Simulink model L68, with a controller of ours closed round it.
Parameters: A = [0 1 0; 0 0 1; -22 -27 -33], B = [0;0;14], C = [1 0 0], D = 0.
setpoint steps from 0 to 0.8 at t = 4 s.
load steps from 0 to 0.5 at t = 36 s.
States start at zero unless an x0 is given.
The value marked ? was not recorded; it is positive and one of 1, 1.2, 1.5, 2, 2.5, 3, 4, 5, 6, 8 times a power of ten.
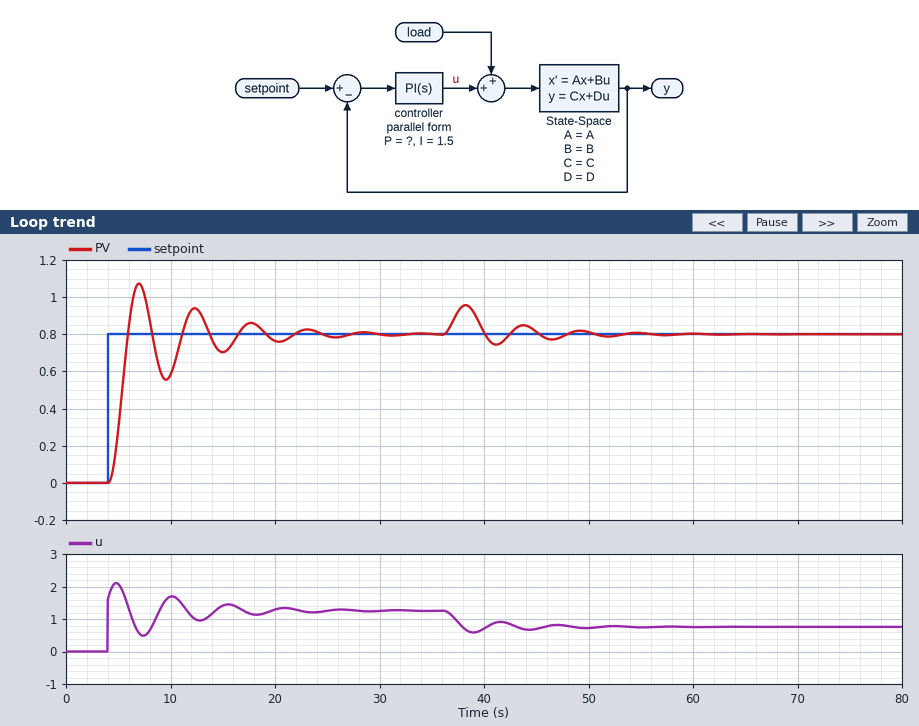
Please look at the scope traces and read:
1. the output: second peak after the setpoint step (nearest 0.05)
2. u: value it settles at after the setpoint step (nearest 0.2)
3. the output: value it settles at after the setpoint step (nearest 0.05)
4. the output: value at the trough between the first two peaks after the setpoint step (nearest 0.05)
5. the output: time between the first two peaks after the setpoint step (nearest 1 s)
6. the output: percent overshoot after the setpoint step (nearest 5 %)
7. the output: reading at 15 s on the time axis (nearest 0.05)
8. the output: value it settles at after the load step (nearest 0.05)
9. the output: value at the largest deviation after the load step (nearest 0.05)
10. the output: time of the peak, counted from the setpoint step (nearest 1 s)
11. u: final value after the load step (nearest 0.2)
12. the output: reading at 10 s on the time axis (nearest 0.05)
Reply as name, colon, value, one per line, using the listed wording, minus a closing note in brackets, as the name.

the output: second peak after the setpoint step: 0.95
u: value it settles at after the setpoint step: 1.2
the output: value it settles at after the setpoint step: 0.80
the output: value at the trough between the first two peaks after the setpoint step: 0.55
the output: time between the first two peaks after the setpoint step: 5 s
the output: percent overshoot after the setpoint step: 35 %
the output: reading at 15 s on the time axis: 0.70
the output: value it settles at after the load step: 0.80
the output: value at the largest deviation after the load step: 0.95
the output: time of the peak, counted from the setpoint step: 3 s
u: final value after the load step: 0.8
the output: reading at 10 s on the time axis: 0.60
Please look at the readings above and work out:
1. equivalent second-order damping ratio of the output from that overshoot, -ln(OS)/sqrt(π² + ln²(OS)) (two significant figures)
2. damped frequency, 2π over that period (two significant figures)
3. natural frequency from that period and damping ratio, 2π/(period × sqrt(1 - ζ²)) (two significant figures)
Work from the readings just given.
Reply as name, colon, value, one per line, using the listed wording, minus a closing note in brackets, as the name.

equivalent second-order damping ratio of the output from that overshoot, -ln(OS)/sqrt(π² + ln²(OS)): 0.32
damped frequency, 2π over that period: 1.3 rad/s
natural frequency from that period and damping ratio, 2π/(period × sqrt(1 - ζ²)): 1.3 rad/s
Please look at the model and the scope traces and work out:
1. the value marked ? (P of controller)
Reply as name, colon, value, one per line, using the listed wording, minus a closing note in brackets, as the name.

the value marked ?: 2
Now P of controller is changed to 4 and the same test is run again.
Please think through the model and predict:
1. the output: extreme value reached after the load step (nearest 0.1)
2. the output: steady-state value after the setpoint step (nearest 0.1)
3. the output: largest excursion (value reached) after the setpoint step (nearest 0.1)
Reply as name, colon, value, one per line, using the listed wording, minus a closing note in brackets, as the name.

the output: extreme value reached after the load step: 0.9
the output: steady-state value after the setpoint step: 0.8
the output: largest excursion (value reached) after the setpoint step: 1.1
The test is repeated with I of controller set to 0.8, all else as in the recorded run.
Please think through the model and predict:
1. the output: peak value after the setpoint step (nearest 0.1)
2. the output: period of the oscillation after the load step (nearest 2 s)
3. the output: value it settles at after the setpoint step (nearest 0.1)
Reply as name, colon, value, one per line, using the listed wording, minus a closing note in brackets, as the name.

the output: peak value after the setpoint step: 0.9
the output: period of the oscillation after the load step: 6 s
the output: value it settles at after the setpoint step: 0.8
